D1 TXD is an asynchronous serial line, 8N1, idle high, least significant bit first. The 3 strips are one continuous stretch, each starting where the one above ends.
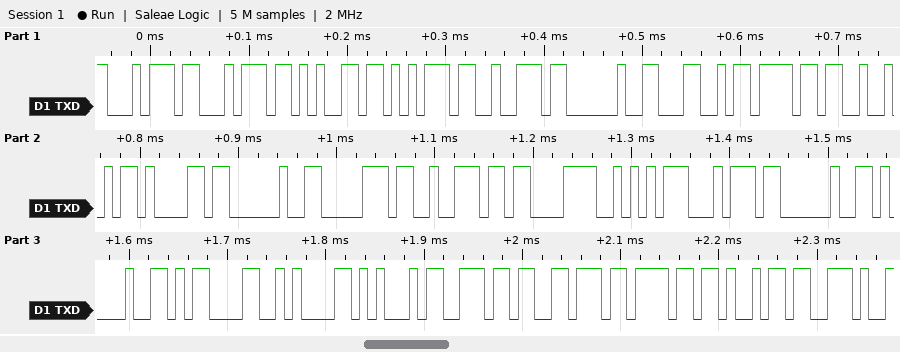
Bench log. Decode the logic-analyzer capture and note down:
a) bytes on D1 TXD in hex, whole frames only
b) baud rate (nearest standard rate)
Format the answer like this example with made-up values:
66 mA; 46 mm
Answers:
0x74 0x74 0x65 0x75 0x72 0x20 0x4C 0x6F 0x52 0x61 0x20 0x70 0x72 0xC3 0xAA 0x74 0x20 0x21 0x0D 0x0A 0x45 0x6E 0x76 0x6F 0x69 0x2E; 115200 baud
